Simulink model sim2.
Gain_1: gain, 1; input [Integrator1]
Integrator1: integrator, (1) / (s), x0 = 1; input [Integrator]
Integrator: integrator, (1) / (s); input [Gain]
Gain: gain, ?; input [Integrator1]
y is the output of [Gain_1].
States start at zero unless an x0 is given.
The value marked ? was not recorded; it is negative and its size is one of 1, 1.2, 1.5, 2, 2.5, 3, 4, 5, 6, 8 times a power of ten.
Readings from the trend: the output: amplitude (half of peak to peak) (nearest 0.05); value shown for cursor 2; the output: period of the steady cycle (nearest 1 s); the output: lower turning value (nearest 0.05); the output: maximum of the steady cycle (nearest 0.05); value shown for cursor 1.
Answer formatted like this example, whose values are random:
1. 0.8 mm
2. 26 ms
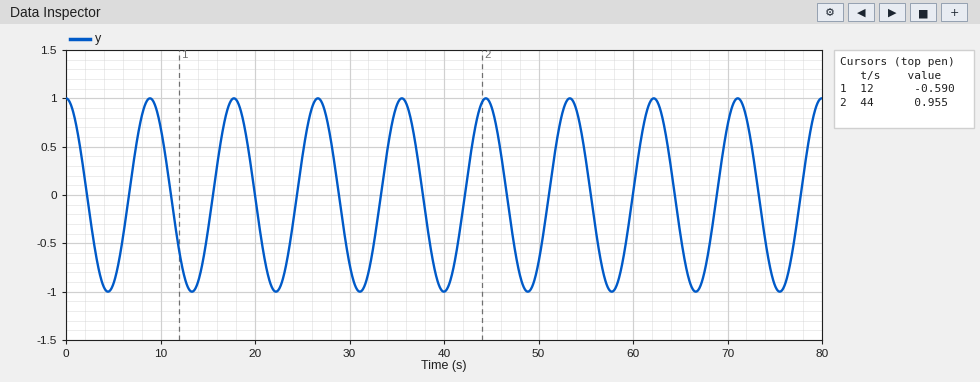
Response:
1. 1.00
2. 0.955
3. 9 s
4. -1.00
5. 1.00
6. -0.590
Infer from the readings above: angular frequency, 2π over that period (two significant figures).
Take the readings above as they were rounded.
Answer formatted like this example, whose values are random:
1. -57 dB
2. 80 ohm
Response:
1. 0.70 rad/s
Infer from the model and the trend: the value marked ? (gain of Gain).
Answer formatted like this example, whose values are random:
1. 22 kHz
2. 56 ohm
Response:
1. -0.5
